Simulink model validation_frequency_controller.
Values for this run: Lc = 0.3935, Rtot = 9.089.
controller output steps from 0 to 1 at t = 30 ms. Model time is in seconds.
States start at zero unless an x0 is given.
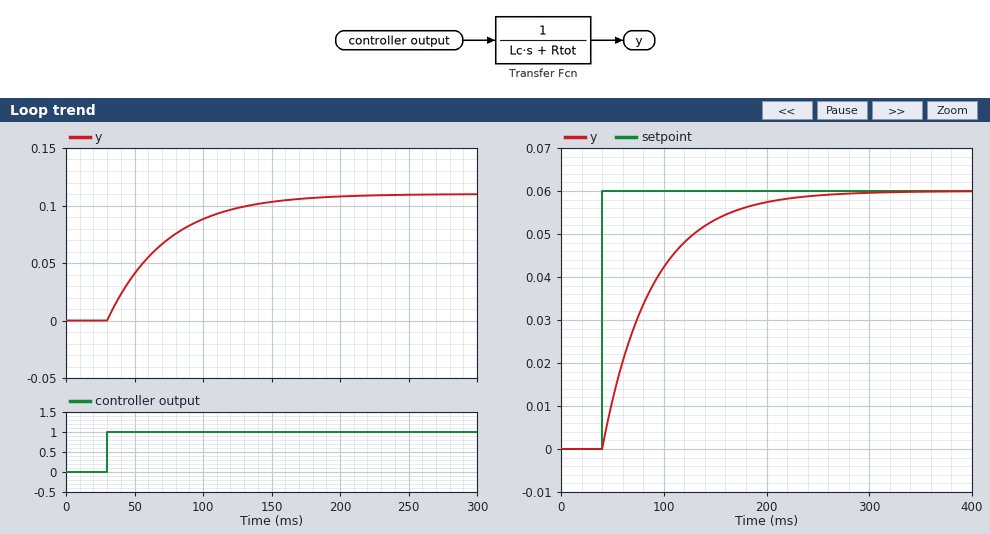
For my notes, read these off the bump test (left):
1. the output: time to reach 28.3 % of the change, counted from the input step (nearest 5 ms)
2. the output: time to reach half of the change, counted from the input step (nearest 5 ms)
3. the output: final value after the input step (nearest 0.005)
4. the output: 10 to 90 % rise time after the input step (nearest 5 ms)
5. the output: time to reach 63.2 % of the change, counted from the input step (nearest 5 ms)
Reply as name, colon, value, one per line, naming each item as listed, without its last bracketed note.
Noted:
the output: time to reach 28.3 % of the change, counted from the input step: 15 ms
the output: time to reach half of the change, counted from the input step: 30 ms
the output: final value after the input step: 0.110
the output: 10 to 90 % rise time after the input step: 95 ms
the output: time to reach 63.2 % of the change, counted from the input step: 45 ms
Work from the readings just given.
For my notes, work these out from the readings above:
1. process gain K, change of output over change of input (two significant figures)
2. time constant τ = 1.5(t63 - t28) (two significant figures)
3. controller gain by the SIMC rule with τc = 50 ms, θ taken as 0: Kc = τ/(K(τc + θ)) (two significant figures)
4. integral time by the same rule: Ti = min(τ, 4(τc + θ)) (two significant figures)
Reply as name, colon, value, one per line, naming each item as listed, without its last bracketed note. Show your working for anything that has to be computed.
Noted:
process gain K, change of output over change of input: (0.11 - 0) / 1 = 0.11
time constant τ = 1.5(t63 - t28): 1.5 × (45 - 15) = 45 ms
controller gain by the SIMC rule with τc = 50 ms, θ taken as 0: Kc = τ/(K(τc + θ)): 45 / (0.11 × (50 + 0)) = 8.2
integral time by the same rule: Ti = min(τ, 4(τc + θ)): min(45, 4 × (50 + 0)) = 45 ms
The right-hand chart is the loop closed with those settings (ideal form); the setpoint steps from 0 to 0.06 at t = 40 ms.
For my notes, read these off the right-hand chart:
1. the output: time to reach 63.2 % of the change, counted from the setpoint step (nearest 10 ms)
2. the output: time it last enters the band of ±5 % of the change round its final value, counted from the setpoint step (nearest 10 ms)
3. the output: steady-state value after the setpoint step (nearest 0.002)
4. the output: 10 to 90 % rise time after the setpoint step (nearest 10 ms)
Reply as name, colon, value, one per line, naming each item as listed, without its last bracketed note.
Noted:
the output: time to reach 63.2 % of the change, counted from the setpoint step: 50 ms
the output: time it last enters the band of ±5 % of the change round its final value, counted from the setpoint step: 150 ms
the output: steady-state value after the setpoint step: 0.060
the output: 10 to 90 % rise time after the setpoint step: 110 ms
